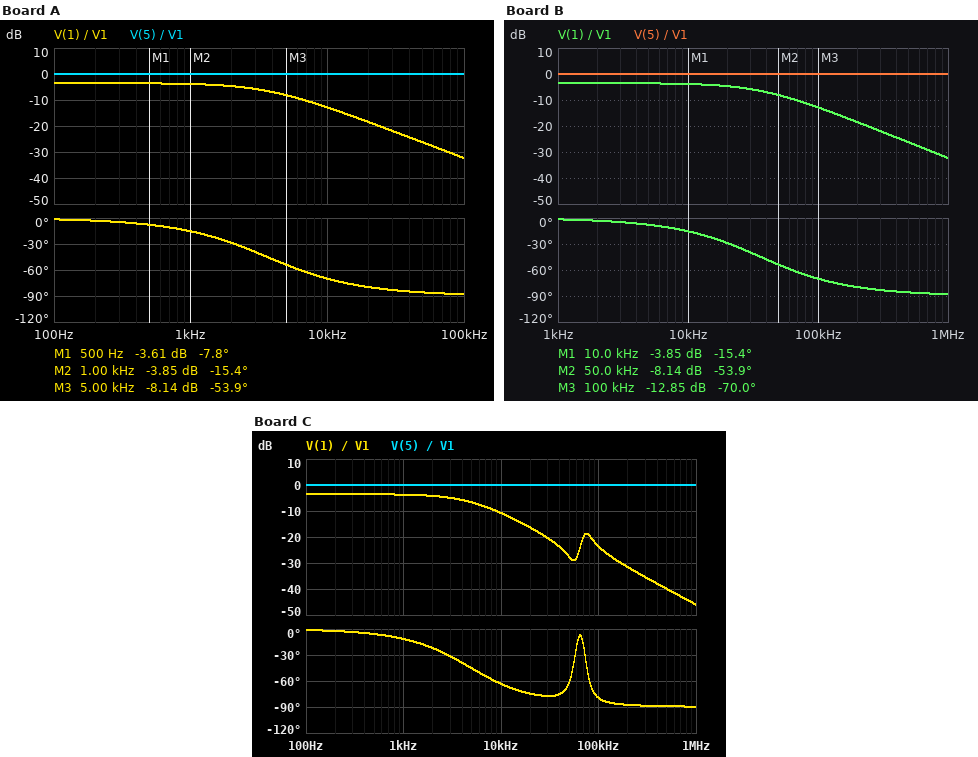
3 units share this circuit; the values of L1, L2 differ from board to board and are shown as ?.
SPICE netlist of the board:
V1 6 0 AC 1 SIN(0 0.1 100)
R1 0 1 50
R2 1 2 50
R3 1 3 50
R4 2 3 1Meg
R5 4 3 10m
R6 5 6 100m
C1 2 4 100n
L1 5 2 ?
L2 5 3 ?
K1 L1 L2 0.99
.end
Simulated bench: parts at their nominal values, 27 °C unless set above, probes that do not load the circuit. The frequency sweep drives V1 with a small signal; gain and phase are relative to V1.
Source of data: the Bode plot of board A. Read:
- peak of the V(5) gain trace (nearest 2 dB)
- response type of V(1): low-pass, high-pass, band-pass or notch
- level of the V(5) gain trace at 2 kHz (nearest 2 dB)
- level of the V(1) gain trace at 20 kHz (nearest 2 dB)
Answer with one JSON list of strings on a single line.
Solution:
["0 dB", "low-pass", "0 dB", "-18 dB"]
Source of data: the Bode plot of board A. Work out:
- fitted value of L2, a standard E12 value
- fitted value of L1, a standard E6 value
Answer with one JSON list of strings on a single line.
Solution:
["3.3 mH", "3.3 mH"]
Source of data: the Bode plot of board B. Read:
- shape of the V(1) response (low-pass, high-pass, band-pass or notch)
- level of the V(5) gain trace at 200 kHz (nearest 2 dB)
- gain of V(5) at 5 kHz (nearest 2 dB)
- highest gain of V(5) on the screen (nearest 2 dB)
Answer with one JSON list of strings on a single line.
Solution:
["low-pass", "0 dB", "0 dB", "0 dB"]
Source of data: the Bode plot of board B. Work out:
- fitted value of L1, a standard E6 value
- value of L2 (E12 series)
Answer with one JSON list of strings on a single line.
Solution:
["330 µH", "330 µH"]
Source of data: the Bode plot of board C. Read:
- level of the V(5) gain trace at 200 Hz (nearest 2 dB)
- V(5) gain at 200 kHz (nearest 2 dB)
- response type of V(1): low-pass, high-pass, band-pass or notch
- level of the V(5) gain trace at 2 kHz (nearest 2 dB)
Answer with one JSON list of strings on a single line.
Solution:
["0 dB", "0 dB", "low-pass", "0 dB"]
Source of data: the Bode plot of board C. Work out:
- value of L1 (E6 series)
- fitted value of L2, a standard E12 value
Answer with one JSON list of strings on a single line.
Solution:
["2.2 mH", "2.7 mH"]
